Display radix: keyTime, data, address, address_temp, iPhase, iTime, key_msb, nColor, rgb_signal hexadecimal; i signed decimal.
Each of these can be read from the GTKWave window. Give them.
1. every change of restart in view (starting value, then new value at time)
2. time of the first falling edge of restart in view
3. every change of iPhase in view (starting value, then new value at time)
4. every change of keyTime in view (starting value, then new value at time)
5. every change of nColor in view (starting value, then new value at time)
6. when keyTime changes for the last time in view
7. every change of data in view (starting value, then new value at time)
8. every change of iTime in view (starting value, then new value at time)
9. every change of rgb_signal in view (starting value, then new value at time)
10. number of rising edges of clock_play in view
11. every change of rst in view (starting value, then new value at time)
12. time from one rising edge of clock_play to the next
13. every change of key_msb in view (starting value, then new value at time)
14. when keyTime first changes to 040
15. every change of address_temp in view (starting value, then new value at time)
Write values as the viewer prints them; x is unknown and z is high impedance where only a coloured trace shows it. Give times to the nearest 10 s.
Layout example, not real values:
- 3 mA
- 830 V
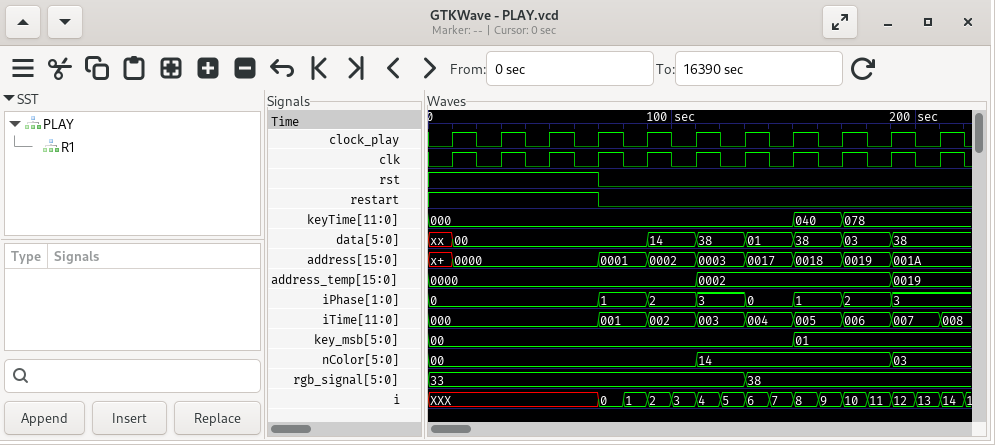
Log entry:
- 1, 0 at 70 s
- 70 s
- 0, 1 at 70 s, 2 at 90 s, 3 at 110 s, 0 at 130 s, 1 at 150 s, 2 at 170 s, 3 at 190 s
- 000, 040 at 150 s, 078 at 170 s
- 00, 14 at 110 s, 03 at 190 s
- 170 s
- xx, 00 at 10 s, 14 at 90 s, 38 at 110 s, 01 at 130 s, 38 at 150 s, 03 at 170 s, 38 at 190 s
- 000, 001 at 70 s, 002 at 90 s, 003 at 110 s, 004 at 130 s, 005 at 150 s, 006 at 170 s, 007 at 190 s, 008 at 210 s
- 33, 38 at 130 s
- 11
- 1, 0 at 70 s
- 20 s
- 00, 01 at 150 s
- 150 s
- 0000, 0002 at 110 s, 0019 at 190 s
